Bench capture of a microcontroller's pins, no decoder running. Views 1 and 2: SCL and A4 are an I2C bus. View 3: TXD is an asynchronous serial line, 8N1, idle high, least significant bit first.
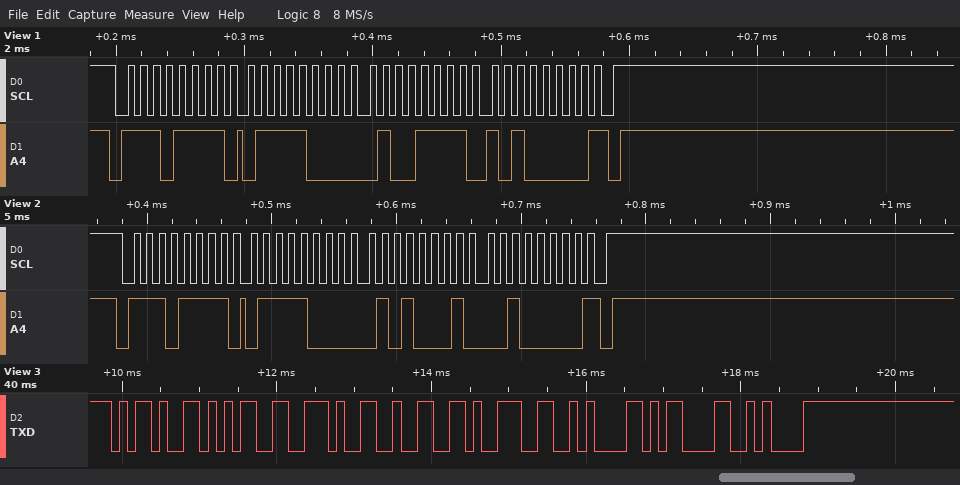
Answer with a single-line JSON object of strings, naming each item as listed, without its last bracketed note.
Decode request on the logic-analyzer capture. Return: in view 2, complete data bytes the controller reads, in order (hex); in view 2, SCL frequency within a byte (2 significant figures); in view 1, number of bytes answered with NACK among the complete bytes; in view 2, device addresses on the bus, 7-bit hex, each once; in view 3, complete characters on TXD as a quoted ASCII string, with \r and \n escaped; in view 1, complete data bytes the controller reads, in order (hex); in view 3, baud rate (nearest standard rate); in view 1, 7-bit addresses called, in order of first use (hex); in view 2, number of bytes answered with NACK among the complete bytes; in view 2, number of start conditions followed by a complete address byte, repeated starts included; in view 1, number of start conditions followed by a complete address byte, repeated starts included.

{"in view 2, complete data bytes the controller reads, in order": "78 51 20", "in view 2, SCL frequency within a byte": "100 kHz", "in view 1, number of bytes answered with NACK among the complete bytes": "1", "in view 2, device addresses on the bus, 7-bit hex, each once": "0x77", "in view 3, complete characters on TXD as a quoted ASCII string, with \\r and \\n escaped": "\"-5.29\\n\\r\\n\"", "in view 1, complete data bytes the controller reads, in order": "78 4F A0", "in view 3, baud rate": "9600 baud", "in view 1, 7-bit addresses called, in order of first use": "0x77", "in view 2, number of bytes answered with NACK among the complete bytes": "1", "in view 2, number of start conditions followed by a complete address byte, repeated starts included": "1", "in view 1, number of start conditions followed by a complete address byte, repeated starts included": "1"}
